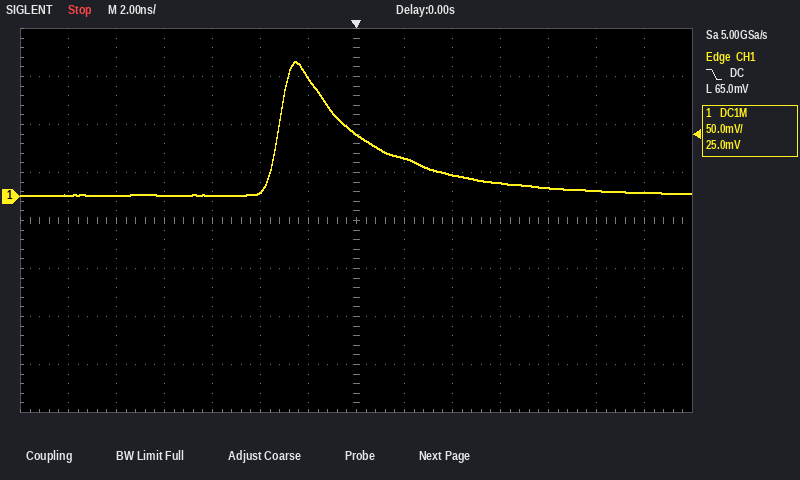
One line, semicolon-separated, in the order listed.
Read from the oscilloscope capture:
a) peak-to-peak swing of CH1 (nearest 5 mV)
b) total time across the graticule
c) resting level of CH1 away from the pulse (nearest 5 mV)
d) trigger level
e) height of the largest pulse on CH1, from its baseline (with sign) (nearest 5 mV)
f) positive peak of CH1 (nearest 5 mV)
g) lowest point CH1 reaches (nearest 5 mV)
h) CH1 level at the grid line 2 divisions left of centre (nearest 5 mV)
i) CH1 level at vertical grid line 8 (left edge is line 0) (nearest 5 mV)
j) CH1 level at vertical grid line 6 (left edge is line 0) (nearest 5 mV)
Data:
140 mV; 28 ns; 0 mV; 65.0 mV; +140 mV; 140 mV; 0 mV; 5 mV; 40 mV; 125 mV
